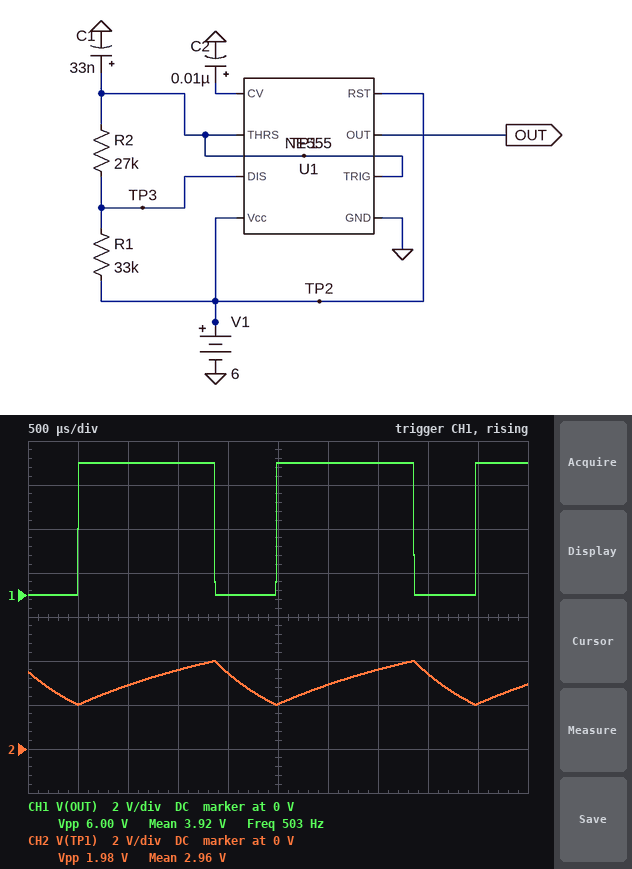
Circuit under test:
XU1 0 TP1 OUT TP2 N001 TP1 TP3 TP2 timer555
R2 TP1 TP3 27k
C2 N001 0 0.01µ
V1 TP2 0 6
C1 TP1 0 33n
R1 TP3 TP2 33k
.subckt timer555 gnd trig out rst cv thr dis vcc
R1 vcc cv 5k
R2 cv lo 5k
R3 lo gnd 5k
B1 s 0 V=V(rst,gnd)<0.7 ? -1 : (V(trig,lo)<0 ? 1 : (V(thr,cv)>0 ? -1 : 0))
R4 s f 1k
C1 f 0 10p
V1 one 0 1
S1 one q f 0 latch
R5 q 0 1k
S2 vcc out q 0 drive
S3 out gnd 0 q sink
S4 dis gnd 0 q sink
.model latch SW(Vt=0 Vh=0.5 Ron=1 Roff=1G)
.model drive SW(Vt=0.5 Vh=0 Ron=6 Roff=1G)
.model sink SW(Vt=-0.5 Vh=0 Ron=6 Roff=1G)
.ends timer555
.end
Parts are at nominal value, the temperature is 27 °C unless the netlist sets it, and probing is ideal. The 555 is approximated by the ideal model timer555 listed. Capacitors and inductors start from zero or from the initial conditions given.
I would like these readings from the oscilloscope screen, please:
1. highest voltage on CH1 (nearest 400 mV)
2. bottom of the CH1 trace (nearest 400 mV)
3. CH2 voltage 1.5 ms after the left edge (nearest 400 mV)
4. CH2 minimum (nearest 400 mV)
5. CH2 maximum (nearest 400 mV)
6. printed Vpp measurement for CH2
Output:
6.0 V
0 V
3.6 V
2.0 V
4.0 V
1.98 V
